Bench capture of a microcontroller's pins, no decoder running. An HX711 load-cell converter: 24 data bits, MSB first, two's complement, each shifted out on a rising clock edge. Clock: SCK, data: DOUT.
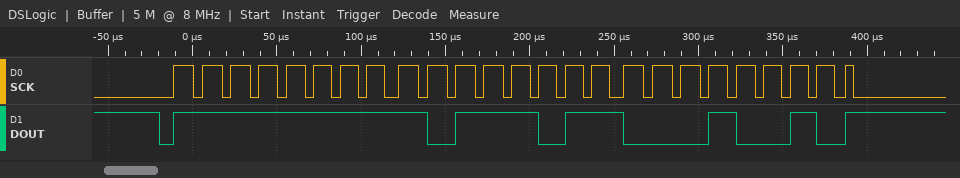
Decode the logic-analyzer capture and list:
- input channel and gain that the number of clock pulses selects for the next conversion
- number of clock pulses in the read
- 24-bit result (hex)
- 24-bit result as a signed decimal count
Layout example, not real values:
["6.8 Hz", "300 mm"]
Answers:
["channel A, gain 128", "25", "0xFFBB12", "-17646"]
